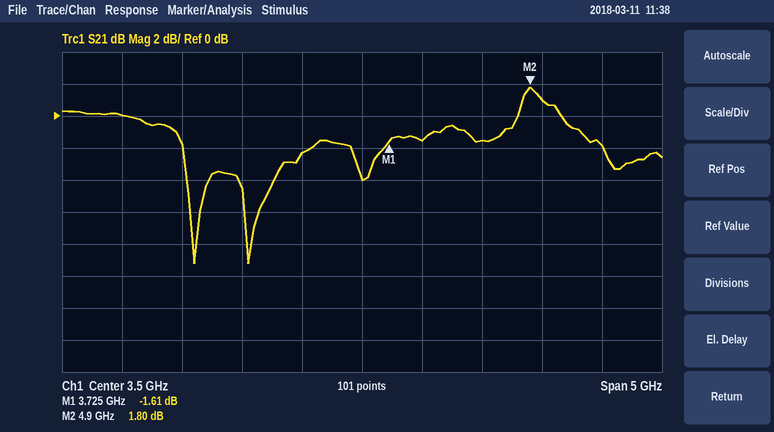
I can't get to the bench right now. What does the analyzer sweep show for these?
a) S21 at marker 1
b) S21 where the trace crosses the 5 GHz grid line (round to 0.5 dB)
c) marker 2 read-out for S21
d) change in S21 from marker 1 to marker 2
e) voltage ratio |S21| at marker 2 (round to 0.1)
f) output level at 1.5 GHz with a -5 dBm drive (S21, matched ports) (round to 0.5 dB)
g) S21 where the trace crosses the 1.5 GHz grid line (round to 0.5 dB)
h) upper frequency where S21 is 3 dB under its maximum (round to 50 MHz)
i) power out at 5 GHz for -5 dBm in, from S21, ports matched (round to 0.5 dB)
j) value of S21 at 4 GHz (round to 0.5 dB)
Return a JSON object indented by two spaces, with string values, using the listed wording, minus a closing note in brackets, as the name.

{
  "S21 at marker 1": "-1.61 dB",
  "S21 where the trace crosses the 5 GHz grid line": "1.0 dB",
  "marker 2 read-out for S21": "1.80 dB",
  "change in S21 from marker 1 to marker 2": "3.41 dB",
  "voltage ratio |S21| at marker 2": "1.2",
  "output level at 1.5 GHz with a -5 dBm drive (S21, matched ports)": "-5.0 dBm",
  "S21 where the trace crosses the 1.5 GHz grid line": "0.0 dB",
  "upper frequency where S21 is 3 dB under its maximum": "5.35 GHz",
  "power out at 5 GHz for -5 dBm in, from S21, ports matched": "-4.0 dBm",
  "value of S21 at 4 GHz": "-1.5 dB"
}
